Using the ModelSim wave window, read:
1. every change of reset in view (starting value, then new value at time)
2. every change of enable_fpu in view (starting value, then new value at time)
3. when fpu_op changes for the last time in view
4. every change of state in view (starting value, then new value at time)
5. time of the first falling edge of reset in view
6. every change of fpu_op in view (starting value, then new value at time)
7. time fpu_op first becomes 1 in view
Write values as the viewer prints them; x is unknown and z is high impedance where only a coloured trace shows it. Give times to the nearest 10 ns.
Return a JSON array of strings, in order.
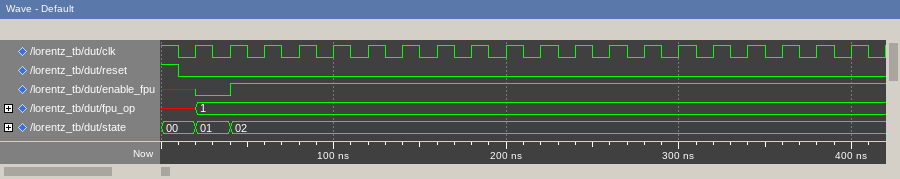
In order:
["1, 0 at 10 ns", "x, 0 at 20 ns, 1 at 40 ns", "20 ns", "00, 01 at 20 ns, 02 at 40 ns", "10 ns", "x, 1 at 20 ns", "20 ns"]
